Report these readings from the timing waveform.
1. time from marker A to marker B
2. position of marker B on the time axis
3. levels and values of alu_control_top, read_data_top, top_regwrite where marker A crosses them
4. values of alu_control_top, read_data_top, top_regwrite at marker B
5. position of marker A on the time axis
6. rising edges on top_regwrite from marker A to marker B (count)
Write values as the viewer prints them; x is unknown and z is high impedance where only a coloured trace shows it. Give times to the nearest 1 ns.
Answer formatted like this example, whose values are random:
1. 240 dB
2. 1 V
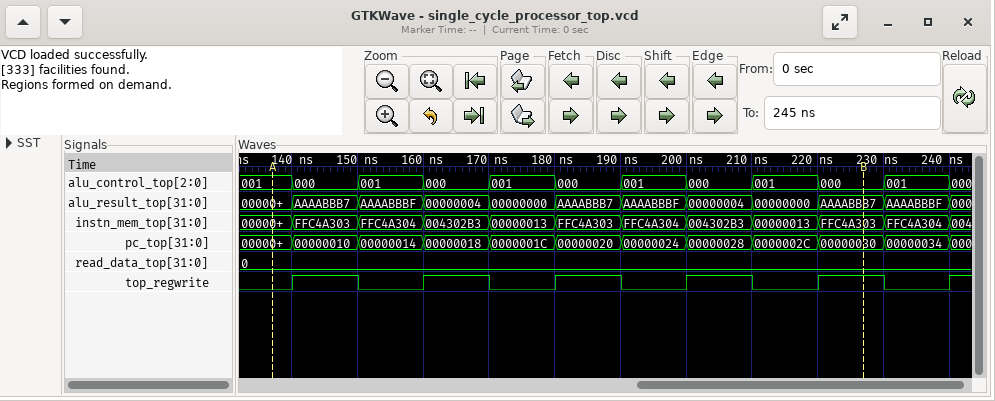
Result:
1. 90 ns
2. 227 ns
3. alu_control_top=001, read_data_top=0, top_regwrite=0
4. alu_control_top=000, read_data_top=0, top_regwrite=1
5. 137 ns
6. 5
